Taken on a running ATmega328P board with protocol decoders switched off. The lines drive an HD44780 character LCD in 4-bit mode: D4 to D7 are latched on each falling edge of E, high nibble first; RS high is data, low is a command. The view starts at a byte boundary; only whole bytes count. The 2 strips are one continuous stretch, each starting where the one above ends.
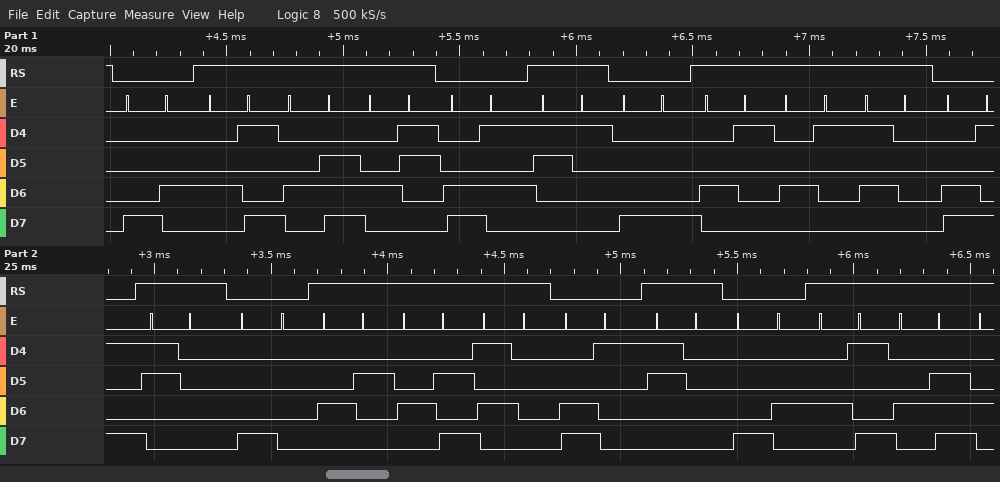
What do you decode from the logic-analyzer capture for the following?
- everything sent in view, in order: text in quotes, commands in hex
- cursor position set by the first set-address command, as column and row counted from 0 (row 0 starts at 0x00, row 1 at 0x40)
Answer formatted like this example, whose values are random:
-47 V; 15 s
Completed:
0x84 "INC" 0xC5 "1" 0x88 "AAP" 0xC9 "0" 0x80 "BJP" 0xC1 "0" 0x84 "IN"; column 4, row 0
